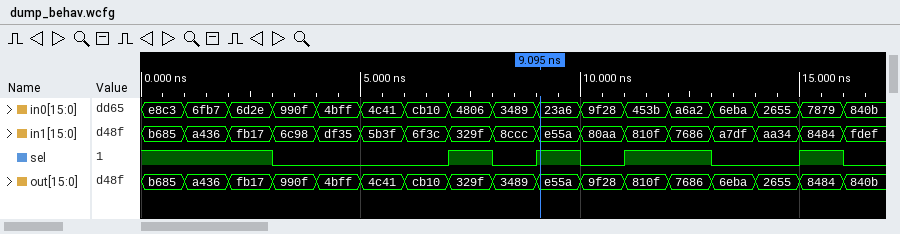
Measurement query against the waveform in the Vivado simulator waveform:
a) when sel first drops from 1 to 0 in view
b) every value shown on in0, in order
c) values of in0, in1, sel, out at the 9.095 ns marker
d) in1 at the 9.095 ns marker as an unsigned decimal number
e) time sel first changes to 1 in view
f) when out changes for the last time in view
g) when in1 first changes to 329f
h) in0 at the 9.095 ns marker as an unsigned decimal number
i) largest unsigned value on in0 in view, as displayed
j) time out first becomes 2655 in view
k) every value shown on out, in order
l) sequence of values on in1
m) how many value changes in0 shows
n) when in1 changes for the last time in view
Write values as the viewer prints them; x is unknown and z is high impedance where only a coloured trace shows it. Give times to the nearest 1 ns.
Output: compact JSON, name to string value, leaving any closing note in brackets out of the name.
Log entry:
{"when sel first drops from 1 to 0 in view": "3 ns", "every value shown on in0, in order": "e8c3, 6fb7, 6d2e, 990f, 4bff, 4c41, cb10, 4806, 3489, 23a6, 9f28, 453b, a6a2, 6eba, 2655, 7879, 840b", "values of in0, in1, sel, out at the 9.095 ns marker": "in0=23a6, in1=e55a, sel=1, out=e55a", "in1 at the 9.095 ns marker as an unsigned decimal number": "58714", "time sel first changes to 1 in view": "7 ns", "when out changes for the last time in view": "16 ns", "when in1 first changes to 329f": "7 ns", "in0 at the 9.095 ns marker as an unsigned decimal number": "9126", "largest unsigned value on in0 in view, as displayed": "e8c3", "time out first becomes 2655 in view": "14 ns", "every value shown on out, in order": "b685, a436, fb17, 990f, 4bff, 4c41, cb10, 329f, 3489, e55a, 9f28, 810f, 7686, 6eba, 2655, 8484, 840b", "sequence of values on in1": "b685, a436, fb17, 6c98, df35, 5b3f, 6f3c, 329f, 8ccc, e55a, 80aa, 810f, 7686, a7df, aa34, 8484, fdef", "how many value changes in0 shows": "16", "when in1 changes for the last time in view": "16 ns"}
